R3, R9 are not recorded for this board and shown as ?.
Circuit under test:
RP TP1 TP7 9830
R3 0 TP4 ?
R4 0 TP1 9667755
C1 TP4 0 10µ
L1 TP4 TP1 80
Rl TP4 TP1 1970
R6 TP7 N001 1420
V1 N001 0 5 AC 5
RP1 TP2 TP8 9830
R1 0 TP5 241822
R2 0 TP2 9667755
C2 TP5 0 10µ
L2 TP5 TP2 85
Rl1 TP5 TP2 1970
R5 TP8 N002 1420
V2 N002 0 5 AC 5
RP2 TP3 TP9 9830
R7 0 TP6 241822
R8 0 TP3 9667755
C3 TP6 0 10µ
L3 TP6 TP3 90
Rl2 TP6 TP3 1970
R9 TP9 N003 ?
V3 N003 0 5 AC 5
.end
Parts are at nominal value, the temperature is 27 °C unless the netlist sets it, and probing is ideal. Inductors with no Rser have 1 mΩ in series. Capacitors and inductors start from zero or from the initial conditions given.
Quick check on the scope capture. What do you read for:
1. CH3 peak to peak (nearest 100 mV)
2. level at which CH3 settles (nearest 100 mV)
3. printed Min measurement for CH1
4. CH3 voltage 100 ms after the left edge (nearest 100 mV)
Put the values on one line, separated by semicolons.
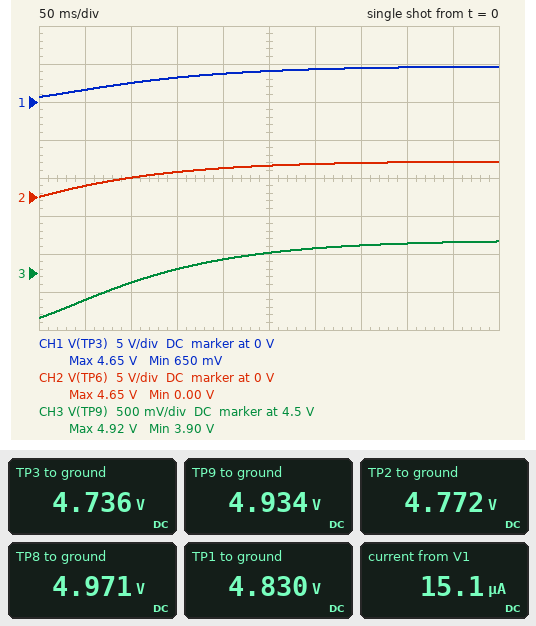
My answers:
1.0 V; 4.9 V; 650 mV; 4.4 V
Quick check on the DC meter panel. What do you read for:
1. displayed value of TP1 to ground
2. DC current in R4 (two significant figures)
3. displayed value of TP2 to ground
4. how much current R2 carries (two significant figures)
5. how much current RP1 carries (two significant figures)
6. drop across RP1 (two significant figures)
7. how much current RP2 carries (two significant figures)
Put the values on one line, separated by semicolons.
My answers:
4.830 V; 500 nA; 4.772 V; 490 nA; 20 µA; 200 mV; 20 µA
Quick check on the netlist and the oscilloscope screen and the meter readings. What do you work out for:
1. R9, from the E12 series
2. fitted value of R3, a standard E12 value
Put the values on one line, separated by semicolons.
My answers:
3.3 kΩ; 330 kΩ
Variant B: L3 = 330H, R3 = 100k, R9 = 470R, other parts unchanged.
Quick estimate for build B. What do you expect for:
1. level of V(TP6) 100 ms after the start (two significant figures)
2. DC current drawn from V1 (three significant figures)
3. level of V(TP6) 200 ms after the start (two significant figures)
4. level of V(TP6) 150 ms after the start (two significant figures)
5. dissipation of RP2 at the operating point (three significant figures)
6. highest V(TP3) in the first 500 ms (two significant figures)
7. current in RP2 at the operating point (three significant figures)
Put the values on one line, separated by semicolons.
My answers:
2.8 V; 45.4 µA; 4.1 V; 3.6 V; 4.05 µW; 4.8 V; 20.3 µA
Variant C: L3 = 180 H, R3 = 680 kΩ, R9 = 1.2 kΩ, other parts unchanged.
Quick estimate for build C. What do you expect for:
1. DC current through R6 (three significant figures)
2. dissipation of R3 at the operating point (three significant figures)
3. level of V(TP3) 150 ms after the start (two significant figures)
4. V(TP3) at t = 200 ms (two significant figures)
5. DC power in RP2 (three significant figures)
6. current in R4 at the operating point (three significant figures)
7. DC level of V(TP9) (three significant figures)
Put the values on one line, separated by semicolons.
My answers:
7.73 µA; 35.5 µW; 3.5 V; 3.9 V; 4.03 µW; 508 nA; 4.98 V
